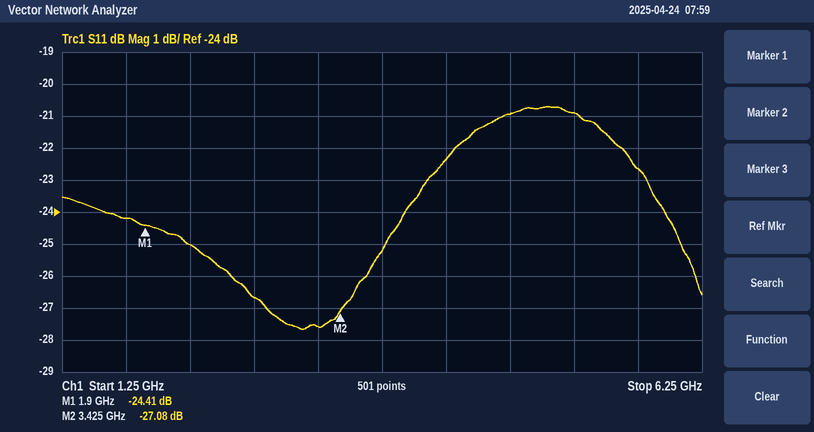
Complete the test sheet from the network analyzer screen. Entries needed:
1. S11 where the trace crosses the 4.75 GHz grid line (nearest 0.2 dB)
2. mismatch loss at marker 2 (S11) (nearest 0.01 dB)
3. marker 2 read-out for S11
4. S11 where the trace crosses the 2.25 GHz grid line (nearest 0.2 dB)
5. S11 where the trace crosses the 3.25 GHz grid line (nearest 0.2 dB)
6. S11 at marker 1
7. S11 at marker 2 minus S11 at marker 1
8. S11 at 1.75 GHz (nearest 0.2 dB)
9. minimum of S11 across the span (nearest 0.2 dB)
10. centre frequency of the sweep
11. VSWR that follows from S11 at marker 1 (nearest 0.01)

-21.0 dB
0.01 dB
-27.08 dB
-25.0 dB
-27.6 dB
-24.41 dB
-2.67 dB
-24.2 dB
-27.6 dB
3.75 GHz
1.13
